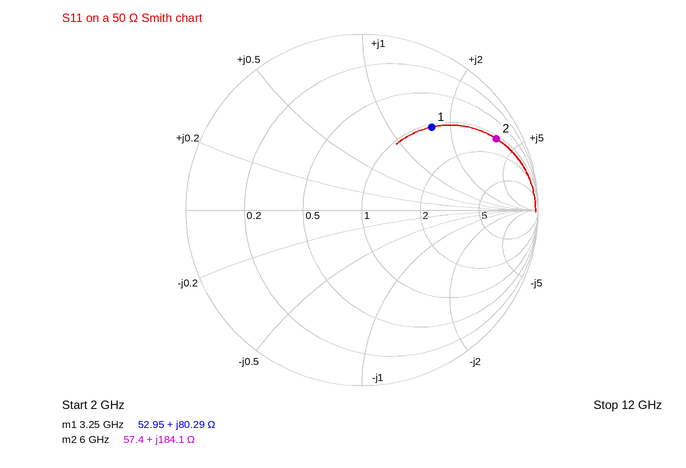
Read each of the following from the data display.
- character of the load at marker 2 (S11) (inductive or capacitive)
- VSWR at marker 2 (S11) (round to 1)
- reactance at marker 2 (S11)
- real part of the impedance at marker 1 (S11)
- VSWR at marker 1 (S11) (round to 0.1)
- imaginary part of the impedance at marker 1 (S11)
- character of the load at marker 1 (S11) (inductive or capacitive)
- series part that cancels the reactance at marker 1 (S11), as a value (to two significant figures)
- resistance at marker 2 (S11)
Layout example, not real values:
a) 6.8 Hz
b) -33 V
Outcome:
a) inductive
b) 14
c) +184.1 Ω
d) 52.95 Ω
e) 4.2
f) +80.29 Ω
g) inductive
h) 610 fF
i) 57.4 Ω
